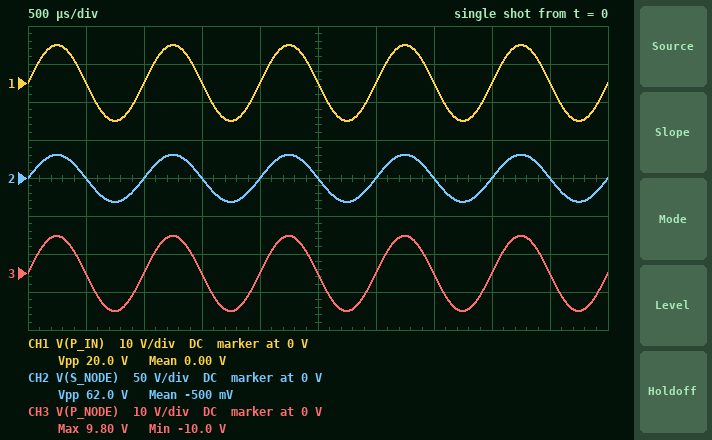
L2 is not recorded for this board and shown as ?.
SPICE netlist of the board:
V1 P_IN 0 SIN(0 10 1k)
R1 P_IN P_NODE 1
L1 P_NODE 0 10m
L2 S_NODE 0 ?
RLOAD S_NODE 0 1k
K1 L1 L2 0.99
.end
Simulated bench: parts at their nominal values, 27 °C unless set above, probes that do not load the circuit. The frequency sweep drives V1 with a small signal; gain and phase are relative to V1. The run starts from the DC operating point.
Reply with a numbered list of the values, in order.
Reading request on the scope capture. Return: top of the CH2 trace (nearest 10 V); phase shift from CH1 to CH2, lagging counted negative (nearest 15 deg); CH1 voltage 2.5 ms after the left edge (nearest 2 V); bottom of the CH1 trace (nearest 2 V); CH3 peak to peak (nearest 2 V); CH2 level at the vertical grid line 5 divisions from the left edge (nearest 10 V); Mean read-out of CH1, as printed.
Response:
1. 30 V
2. 0 deg
3. 0 V
4. -10 V
5. 20 V
6. 0 V
7. 0.00 V
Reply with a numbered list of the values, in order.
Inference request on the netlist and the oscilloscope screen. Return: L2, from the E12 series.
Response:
1. 100 mH
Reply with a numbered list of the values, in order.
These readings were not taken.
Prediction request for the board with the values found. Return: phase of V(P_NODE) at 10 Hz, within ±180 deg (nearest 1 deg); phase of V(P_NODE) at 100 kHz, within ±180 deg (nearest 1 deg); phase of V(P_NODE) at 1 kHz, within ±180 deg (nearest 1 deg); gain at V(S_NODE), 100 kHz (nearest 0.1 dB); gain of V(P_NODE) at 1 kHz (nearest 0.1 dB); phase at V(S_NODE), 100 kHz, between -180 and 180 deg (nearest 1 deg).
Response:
1. 58 deg
2. 0 deg
3. 1 deg
4. 5.8 dB
5. -0.1 dB
6. -51 deg
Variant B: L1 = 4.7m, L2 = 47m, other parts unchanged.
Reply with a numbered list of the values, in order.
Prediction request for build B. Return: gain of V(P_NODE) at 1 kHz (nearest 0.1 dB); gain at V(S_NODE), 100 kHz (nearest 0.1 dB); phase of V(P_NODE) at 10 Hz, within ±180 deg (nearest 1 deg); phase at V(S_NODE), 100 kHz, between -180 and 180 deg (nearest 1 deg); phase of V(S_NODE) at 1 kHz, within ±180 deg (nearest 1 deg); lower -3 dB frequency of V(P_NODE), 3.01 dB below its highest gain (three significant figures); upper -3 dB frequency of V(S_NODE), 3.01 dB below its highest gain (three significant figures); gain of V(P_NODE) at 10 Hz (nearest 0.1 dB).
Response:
1. -0.1 dB
2. 8.6 dB
3. 73 deg
4. -30 deg
5. 2 deg
6. 34.2 Hz
7. 172 kHz
8. -11.0 dB
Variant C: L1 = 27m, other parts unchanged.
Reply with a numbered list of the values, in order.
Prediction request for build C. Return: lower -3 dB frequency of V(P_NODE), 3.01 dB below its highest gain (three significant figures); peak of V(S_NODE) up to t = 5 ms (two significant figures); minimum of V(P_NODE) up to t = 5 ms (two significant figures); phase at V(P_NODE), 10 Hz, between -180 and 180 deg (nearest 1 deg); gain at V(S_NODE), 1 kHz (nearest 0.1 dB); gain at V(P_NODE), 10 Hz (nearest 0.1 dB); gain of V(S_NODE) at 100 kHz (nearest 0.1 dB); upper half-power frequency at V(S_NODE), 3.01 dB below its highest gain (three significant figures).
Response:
1. 5.92 Hz
2. 19 V
3. -10 V
4. 30 deg
5. 5.6 dB
6. -1.3 dB
7. 1.5 dB
8. 80.3 kHz
